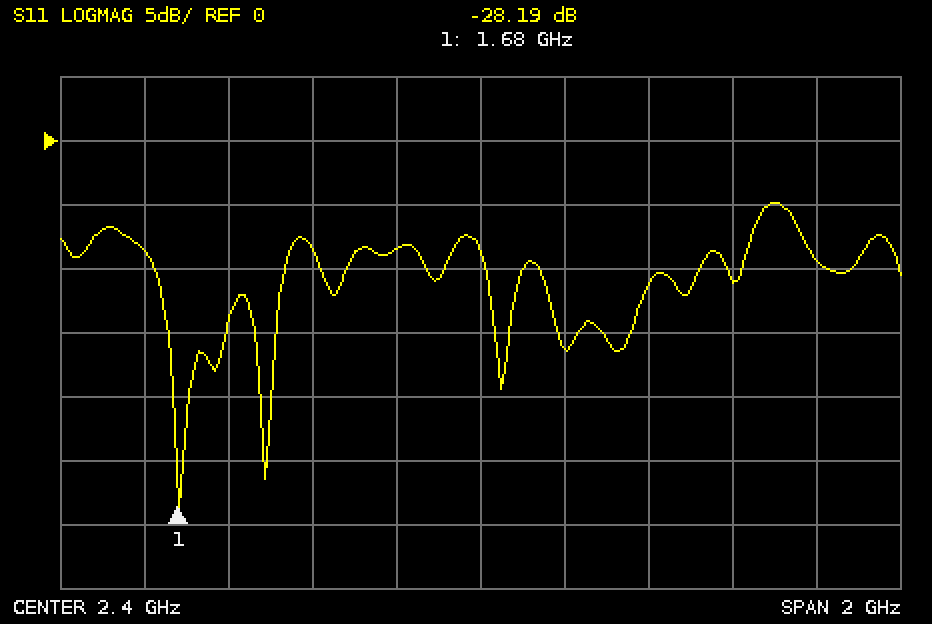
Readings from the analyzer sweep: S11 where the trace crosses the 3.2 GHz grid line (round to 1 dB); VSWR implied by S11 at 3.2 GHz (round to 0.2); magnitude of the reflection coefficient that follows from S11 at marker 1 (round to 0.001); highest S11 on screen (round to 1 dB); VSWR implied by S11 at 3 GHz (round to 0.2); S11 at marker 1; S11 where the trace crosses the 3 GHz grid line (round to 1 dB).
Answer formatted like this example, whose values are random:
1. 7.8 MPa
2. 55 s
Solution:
1. -9 dB
2. 2.0
3. 0.039
4. -5 dB
5. 1.8
6. -28.19 dB
7. -11 dB
